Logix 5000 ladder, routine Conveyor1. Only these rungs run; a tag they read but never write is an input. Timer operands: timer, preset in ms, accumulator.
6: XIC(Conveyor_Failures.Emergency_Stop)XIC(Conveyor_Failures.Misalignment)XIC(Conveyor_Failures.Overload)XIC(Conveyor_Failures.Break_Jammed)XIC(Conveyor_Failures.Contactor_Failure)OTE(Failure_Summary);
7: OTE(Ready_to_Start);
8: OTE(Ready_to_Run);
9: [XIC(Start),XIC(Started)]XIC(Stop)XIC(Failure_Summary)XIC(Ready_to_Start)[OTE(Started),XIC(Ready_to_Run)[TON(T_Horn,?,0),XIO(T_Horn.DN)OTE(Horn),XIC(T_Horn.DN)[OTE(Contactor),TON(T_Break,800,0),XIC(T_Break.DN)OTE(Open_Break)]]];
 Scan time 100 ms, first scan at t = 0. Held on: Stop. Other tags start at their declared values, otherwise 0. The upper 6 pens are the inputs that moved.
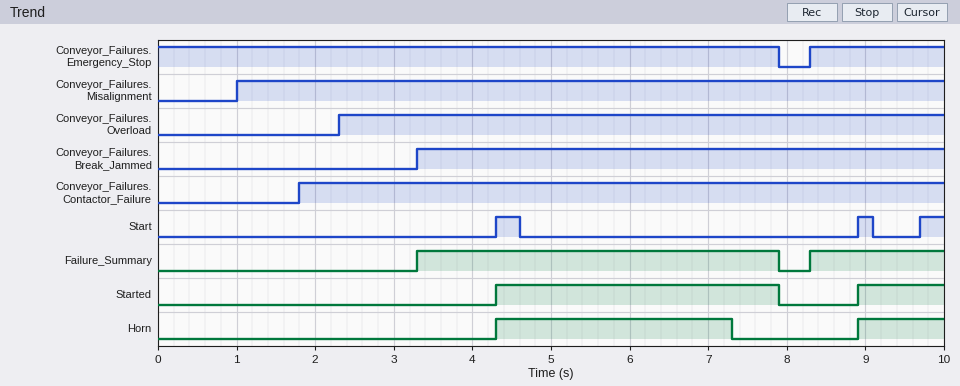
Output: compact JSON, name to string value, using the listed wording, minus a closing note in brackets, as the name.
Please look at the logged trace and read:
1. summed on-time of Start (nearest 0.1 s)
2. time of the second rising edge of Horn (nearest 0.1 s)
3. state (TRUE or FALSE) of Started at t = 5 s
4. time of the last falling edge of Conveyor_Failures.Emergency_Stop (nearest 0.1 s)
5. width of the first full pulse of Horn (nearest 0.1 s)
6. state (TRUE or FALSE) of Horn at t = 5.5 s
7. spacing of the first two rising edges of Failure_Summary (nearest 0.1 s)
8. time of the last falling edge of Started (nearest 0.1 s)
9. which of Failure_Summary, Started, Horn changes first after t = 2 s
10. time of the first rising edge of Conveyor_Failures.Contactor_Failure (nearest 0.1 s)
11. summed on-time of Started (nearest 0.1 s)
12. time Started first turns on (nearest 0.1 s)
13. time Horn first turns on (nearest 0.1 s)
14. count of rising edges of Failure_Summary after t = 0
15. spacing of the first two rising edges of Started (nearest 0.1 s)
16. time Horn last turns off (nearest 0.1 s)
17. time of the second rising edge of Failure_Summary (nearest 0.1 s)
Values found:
{"summed on-time of Start": "0.8 s", "time of the second rising edge of Horn": "8.9 s", "state (TRUE or FALSE) of Started at t = 5 s": "TRUE", "time of the last falling edge of Conveyor_Failures.Emergency_Stop": "7.9 s", "width of the first full pulse of Horn": "3.0 s", "state (TRUE or FALSE) of Horn at t = 5.5 s": "TRUE", "spacing of the first two rising edges of Failure_Summary": "5.0 s", "time of the last falling edge of Started": "7.9 s", "which of Failure_Summary, Started, Horn changes first after t = 2 s": "Failure_Summary", "time of the first rising edge of Conveyor_Failures.Contactor_Failure": "1.8 s", "summed on-time of Started": "4.7 s", "time Started first turns on": "4.3 s", "time Horn first turns on": "4.3 s", "count of rising edges of Failure_Summary after t = 0": "2", "spacing of the first two rising edges of Started": "4.6 s", "time Horn last turns off": "7.3 s", "time of the second rising edge of Failure_Summary": "8.3 s"}
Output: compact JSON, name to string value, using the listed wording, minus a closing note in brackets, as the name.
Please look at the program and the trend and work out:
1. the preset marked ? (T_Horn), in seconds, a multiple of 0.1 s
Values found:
{"the preset marked ? (T_Horn), in seconds, a multiple of 0.1 s": "3.0 s"}
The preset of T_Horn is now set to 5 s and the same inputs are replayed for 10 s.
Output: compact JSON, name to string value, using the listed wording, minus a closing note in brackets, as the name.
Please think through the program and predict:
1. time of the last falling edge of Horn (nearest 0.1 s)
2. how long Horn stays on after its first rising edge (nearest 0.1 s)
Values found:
{"time of the last falling edge of Horn": "7.9 s", "how long Horn stays on after its first rising edge": "3.6 s"}
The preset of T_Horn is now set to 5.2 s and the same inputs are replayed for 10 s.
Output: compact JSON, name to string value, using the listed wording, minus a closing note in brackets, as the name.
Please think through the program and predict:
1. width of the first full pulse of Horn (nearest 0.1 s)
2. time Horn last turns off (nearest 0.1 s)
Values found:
{"width of the first full pulse of Horn": "3.6 s", "time Horn last turns off": "7.9 s"}
